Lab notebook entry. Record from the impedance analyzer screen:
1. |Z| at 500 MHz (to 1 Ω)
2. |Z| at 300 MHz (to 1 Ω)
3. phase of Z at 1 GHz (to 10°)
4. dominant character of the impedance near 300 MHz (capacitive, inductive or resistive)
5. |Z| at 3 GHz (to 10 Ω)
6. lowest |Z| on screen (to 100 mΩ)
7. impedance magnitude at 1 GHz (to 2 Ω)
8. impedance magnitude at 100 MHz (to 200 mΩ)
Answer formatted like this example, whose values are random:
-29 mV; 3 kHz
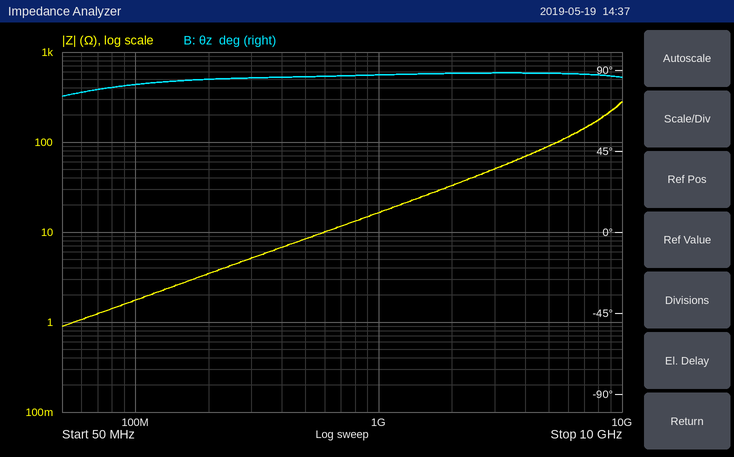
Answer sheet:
8 Ω; 5 Ω; 90°; inductive; 50 Ω; 900 mΩ; 16 Ω; 1.8 Ω
